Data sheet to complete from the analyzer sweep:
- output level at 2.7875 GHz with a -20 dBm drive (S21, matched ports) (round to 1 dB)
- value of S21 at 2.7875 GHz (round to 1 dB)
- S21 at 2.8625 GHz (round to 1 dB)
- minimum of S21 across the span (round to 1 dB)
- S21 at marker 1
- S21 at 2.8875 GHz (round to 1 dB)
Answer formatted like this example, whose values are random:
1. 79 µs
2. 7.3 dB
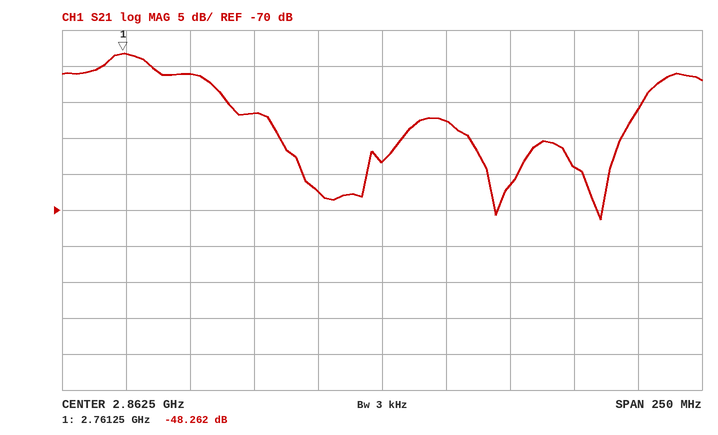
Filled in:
1. -71 dBm
2. -51 dB
3. -63 dB
4. -71 dB
5. -48.262 dB
6. -58 dB
